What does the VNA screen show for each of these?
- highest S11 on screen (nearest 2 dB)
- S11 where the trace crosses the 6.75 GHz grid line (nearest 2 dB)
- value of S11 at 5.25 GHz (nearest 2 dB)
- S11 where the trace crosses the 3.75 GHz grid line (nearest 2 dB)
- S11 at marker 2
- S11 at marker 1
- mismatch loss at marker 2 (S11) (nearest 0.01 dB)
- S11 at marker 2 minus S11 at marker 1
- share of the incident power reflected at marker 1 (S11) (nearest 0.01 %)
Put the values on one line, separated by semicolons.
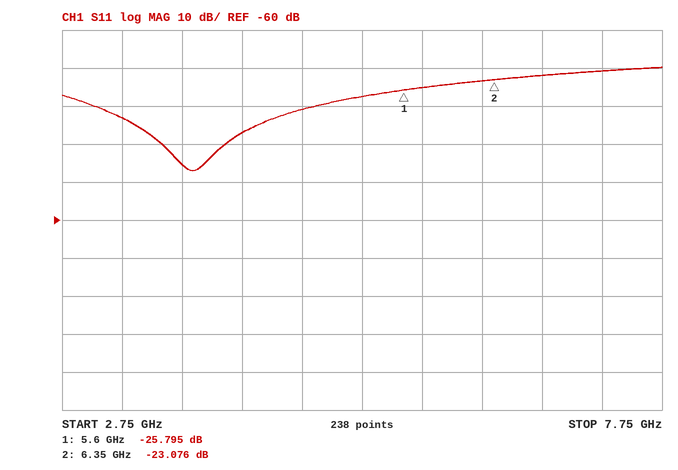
-20 dB; -22 dB; -28 dB; -46 dB; -23.076 dB; -25.795 dB; 0.02 dB; 2.719 dB; 0.26 %
